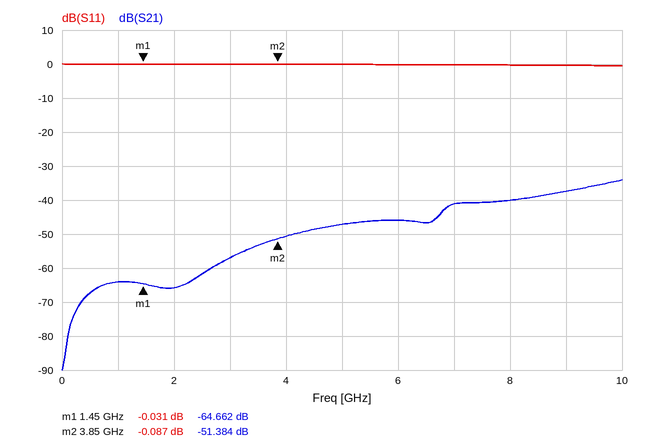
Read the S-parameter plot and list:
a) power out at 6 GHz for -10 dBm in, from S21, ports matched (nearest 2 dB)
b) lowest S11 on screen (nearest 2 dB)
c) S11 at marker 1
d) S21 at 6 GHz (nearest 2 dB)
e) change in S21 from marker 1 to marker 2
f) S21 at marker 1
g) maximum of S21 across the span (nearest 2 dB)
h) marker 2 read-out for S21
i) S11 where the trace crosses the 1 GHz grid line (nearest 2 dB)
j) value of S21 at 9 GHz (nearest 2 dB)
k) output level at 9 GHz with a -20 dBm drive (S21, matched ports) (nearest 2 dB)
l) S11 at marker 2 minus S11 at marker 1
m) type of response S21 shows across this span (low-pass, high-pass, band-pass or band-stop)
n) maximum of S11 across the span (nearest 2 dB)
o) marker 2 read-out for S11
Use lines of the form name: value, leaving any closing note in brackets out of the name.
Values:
power out at 6 GHz for -10 dBm in, from S21, ports matched: -56 dBm
lowest S11 on screen: 0 dB
S11 at marker 1: -0.031 dB
S21 at 6 GHz: -46 dB
change in S21 from marker 1 to marker 2: 13.278 dB
S21 at marker 1: -64.662 dB
maximum of S21 across the span: -34 dB
marker 2 read-out for S21: -51.384 dB
S11 where the trace crosses the 1 GHz grid line: 0 dB
value of S21 at 9 GHz: -38 dB
output level at 9 GHz with a -20 dBm drive (S21, matched ports): -58 dBm
S11 at marker 2 minus S11 at marker 1: -0.056 dB
type of response S21 shows across this span: high-pass
maximum of S11 across the span: 0 dB
marker 2 read-out for S11: -0.087 dB
